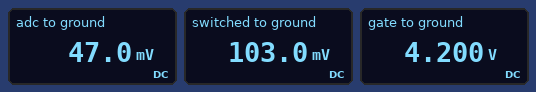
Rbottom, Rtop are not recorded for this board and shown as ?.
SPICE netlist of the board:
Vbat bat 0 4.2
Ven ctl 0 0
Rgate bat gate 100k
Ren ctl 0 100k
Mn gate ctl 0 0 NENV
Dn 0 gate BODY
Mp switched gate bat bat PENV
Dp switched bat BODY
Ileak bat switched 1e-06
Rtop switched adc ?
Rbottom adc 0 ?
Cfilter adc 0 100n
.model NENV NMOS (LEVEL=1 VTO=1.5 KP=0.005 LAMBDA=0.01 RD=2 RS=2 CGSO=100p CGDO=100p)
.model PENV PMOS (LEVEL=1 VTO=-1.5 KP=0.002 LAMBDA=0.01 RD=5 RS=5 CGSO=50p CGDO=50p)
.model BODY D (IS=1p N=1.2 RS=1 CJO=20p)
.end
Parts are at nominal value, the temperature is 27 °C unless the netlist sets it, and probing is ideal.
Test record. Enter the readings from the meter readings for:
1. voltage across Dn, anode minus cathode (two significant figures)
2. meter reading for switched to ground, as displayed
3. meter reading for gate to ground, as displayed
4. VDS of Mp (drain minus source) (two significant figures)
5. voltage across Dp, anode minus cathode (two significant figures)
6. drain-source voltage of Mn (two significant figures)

-4.2 V
103.0 mV
4.200 V
-4.1 V
-4.1 V
4.2 V
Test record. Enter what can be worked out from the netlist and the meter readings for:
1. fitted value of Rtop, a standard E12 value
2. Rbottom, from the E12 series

56 kΩ
47 kΩ
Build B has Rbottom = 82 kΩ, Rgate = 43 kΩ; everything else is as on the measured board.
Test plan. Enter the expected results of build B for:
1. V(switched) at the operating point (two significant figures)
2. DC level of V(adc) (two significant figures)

140 mV
82 mV
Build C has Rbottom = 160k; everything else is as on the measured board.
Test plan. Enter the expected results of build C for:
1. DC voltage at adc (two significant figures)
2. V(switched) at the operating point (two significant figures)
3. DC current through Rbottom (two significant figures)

160 mV
220 mV
1.0 µA
